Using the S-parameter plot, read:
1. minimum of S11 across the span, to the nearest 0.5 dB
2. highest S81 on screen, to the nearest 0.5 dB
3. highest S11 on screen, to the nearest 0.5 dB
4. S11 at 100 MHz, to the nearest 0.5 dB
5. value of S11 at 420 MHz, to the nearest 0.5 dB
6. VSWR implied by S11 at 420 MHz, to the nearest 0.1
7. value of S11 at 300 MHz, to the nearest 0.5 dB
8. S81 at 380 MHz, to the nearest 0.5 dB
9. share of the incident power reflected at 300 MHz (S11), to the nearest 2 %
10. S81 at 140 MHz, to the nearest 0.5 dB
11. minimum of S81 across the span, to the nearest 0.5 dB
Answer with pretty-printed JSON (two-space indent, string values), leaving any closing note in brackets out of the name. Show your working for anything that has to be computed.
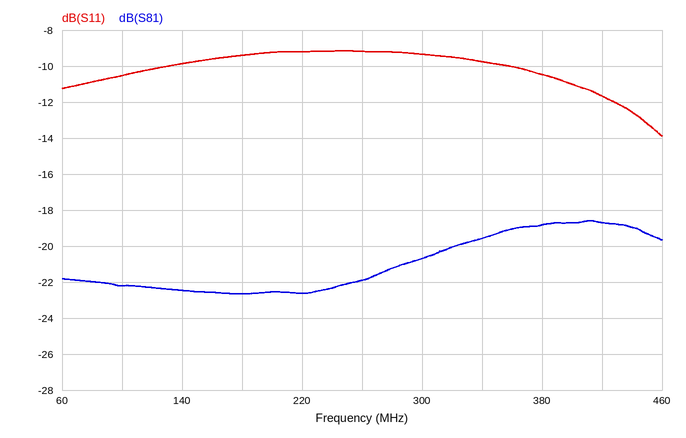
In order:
{
  "minimum of S11 across the span, to the nearest 0.5 dB": "-14.0 dB",
  "highest S81 on screen, to the nearest 0.5 dB": "-18.5 dB",
  "highest S11 on screen, to the nearest 0.5 dB": "-9.0 dB",
  "S11 at 100 MHz, to the nearest 0.5 dB": "-10.5 dB",
  "value of S11 at 420 MHz, to the nearest 0.5 dB": "-11.5 dB",
  "VSWR implied by S11 at 420 MHz, to the nearest 0.1": "|Γ| = 10^(-11.5/20) = 0.2661; VSWR = (1 + 0.2661)/(1 − 0.2661) ≈ 1.7",
  "value of S11 at 300 MHz, to the nearest 0.5 dB": "-9.5 dB",
  "S81 at 380 MHz, to the nearest 0.5 dB": "-19.0 dB",
  "share of the incident power reflected at 300 MHz (S11), to the nearest 2 %": "10^(-9.5/10) ≈ 11.2 %, so 12 % to the nearest 2 %",
  "S81 at 140 MHz, to the nearest 0.5 dB": "-22.5 dB",
  "minimum of S81 across the span, to the nearest 0.5 dB": "-22.5 dB"
}
